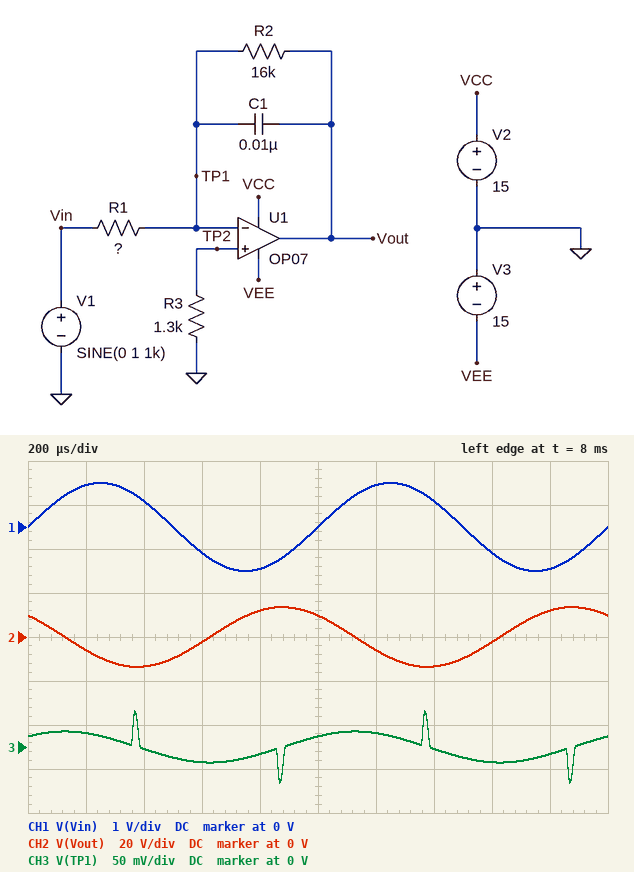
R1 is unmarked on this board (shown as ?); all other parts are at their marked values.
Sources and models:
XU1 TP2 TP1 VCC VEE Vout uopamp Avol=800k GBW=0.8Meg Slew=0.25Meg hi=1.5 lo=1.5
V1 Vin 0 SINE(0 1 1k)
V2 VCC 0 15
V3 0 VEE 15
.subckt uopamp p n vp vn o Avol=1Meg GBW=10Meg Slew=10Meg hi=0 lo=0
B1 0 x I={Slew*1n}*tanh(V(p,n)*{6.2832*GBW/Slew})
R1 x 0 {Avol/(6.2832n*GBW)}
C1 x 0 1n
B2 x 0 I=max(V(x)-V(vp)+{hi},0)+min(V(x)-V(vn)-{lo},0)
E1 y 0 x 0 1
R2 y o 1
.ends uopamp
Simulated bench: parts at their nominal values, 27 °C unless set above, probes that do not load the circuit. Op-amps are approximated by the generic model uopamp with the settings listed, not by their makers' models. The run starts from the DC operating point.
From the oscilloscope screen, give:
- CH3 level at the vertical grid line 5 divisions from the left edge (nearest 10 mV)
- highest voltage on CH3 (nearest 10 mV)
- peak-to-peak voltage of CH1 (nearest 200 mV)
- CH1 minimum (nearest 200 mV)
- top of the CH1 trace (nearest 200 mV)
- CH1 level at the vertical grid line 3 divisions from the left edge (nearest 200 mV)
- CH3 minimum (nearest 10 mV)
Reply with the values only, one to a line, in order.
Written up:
10 mV
40 mV
2.0 V
-1.0 V
1.0 V
-600 mV
-40 mV
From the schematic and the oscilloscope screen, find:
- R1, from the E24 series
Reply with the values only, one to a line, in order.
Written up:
820 Ω
